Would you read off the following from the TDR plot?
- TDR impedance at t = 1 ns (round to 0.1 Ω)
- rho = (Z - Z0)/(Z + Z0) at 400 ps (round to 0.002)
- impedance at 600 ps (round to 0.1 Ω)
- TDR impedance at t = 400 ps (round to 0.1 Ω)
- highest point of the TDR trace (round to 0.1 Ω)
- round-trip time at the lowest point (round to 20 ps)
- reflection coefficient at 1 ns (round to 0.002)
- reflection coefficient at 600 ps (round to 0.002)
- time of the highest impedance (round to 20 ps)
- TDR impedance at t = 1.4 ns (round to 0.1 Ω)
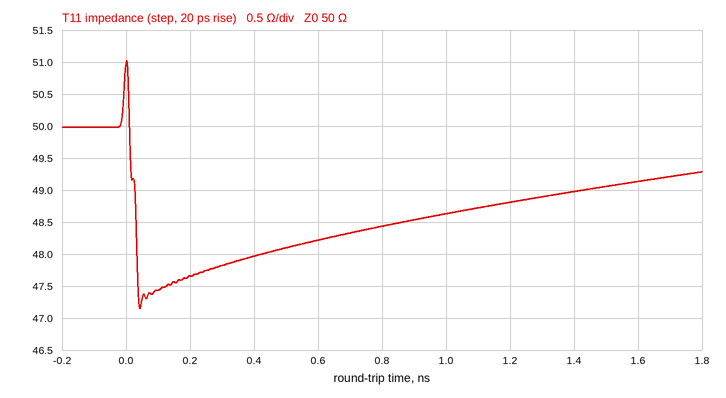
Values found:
48.6 Ω
-0.020
48.2 Ω
48.0 Ω
51.0 Ω
40 ps
-0.014
-0.018
0 ps
49.0 Ω
